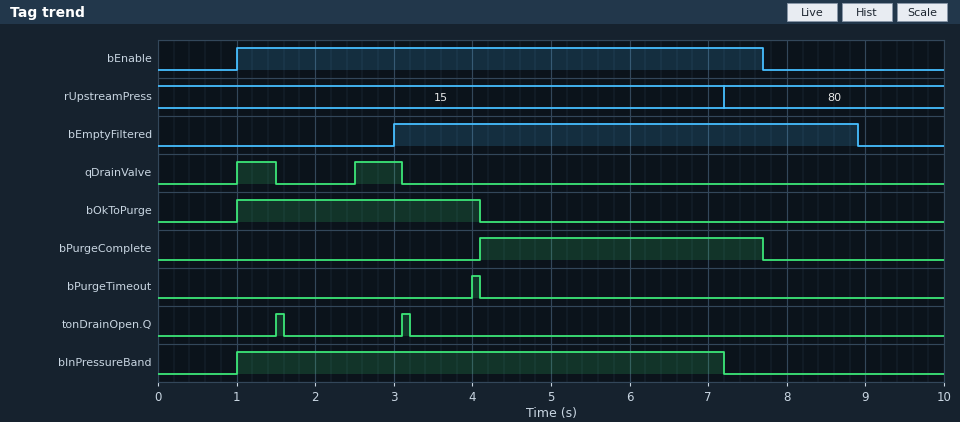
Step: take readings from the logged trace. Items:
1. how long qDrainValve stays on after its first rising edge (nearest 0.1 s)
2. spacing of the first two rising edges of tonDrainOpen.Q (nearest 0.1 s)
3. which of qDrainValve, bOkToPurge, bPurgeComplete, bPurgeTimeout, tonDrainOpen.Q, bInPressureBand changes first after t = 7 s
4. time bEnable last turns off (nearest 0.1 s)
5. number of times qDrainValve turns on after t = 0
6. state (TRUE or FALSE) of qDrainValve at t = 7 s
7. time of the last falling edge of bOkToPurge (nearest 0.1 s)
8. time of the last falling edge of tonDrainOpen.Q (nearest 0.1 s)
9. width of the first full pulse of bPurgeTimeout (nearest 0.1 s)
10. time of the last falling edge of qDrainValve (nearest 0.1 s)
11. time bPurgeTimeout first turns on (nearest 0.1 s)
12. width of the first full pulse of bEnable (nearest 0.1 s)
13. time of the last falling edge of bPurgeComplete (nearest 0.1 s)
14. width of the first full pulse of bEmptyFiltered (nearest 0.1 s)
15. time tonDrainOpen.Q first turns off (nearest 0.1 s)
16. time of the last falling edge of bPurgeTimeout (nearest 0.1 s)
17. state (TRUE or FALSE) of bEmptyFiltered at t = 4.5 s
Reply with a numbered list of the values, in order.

1. 0.5 s
2. 1.6 s
3. bInPressureBand
4. 7.7 s
5. 2
6. FALSE
7. 4.1 s
8. 3.2 s
9. 0.1 s
10. 3.1 s
11. 4.0 s
12. 6.7 s
13. 7.7 s
14. 5.9 s
15. 1.6 s
16. 4.1 s
17. TRUE
